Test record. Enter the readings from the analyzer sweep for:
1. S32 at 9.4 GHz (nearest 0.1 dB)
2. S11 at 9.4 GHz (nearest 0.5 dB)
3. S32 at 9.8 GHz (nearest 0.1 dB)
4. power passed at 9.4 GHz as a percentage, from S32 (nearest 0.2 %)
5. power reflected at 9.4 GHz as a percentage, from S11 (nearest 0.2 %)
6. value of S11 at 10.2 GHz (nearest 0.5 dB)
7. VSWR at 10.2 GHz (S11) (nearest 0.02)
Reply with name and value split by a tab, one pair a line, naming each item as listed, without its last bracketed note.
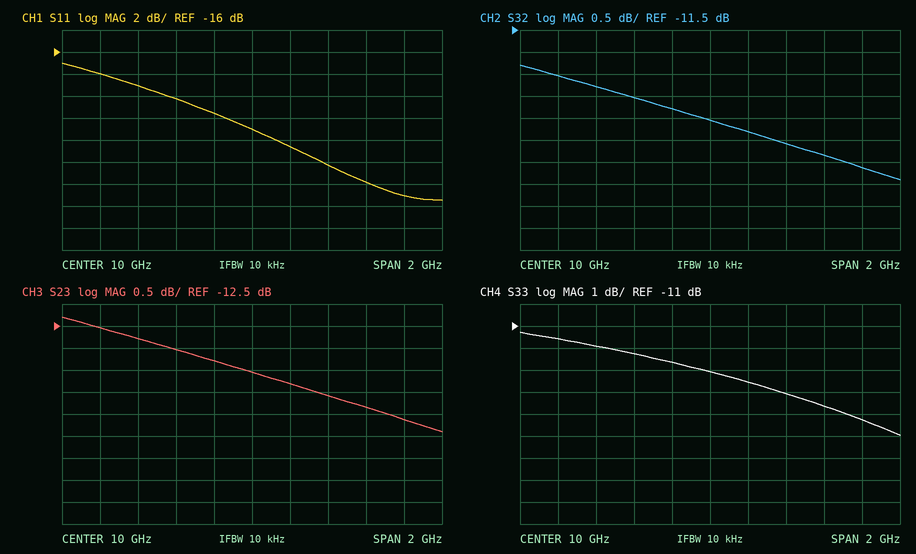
S32 at 9.4 GHz	-12.8 dB
S11 at 9.4 GHz	-19.0 dB
S32 at 9.8 GHz	-13.3 dB
power passed at 9.4 GHz as a percentage, from S32	5.2 %
power reflected at 9.4 GHz as a percentage, from S11	1.2 %
value of S11 at 10.2 GHz	-24.5 dB
VSWR at 10.2 GHz (S11)	1.12
